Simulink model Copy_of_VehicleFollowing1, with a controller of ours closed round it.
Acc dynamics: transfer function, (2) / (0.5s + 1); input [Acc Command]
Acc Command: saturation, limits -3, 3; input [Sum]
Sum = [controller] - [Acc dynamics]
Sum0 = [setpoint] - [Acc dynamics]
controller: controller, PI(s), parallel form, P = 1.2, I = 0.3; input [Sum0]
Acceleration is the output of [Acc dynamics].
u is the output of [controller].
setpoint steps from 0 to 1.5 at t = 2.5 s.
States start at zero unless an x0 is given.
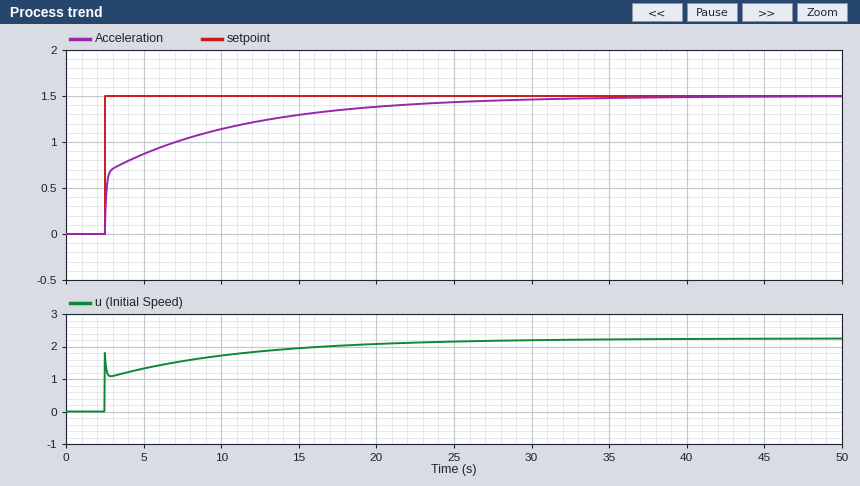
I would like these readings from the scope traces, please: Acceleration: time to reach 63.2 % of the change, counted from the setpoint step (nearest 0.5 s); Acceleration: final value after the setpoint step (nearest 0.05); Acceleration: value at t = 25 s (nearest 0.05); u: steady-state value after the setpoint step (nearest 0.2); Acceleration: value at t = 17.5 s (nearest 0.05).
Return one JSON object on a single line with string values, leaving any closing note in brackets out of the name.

{"Acceleration: time to reach 63.2 % of the change, counted from the setpoint step": "3.5 s", "Acceleration: final value after the setpoint step": "1.50", "Acceleration: value at t = 25 s": "1.45", "u: steady-state value after the setpoint step": "2.2", "Acceleration: value at t = 17.5 s": "1.35"}
